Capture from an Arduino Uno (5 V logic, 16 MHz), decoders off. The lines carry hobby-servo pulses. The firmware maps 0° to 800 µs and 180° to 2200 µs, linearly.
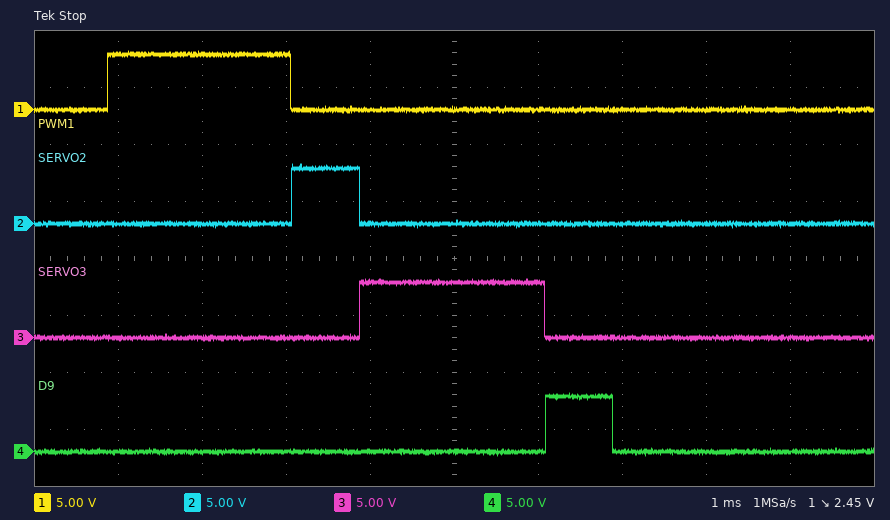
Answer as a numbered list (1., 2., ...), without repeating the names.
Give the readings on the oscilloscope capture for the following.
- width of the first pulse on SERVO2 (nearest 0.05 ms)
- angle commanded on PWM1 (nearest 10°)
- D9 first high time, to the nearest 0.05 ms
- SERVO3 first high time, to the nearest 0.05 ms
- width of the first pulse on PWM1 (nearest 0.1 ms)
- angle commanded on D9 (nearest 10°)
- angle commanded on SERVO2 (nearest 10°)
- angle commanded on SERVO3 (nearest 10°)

1. 0.80 ms
2. 180°
3. 0.80 ms
4. 2.20 ms
5. 2.2 ms
6. 0°
7. 0°
8. 180°
